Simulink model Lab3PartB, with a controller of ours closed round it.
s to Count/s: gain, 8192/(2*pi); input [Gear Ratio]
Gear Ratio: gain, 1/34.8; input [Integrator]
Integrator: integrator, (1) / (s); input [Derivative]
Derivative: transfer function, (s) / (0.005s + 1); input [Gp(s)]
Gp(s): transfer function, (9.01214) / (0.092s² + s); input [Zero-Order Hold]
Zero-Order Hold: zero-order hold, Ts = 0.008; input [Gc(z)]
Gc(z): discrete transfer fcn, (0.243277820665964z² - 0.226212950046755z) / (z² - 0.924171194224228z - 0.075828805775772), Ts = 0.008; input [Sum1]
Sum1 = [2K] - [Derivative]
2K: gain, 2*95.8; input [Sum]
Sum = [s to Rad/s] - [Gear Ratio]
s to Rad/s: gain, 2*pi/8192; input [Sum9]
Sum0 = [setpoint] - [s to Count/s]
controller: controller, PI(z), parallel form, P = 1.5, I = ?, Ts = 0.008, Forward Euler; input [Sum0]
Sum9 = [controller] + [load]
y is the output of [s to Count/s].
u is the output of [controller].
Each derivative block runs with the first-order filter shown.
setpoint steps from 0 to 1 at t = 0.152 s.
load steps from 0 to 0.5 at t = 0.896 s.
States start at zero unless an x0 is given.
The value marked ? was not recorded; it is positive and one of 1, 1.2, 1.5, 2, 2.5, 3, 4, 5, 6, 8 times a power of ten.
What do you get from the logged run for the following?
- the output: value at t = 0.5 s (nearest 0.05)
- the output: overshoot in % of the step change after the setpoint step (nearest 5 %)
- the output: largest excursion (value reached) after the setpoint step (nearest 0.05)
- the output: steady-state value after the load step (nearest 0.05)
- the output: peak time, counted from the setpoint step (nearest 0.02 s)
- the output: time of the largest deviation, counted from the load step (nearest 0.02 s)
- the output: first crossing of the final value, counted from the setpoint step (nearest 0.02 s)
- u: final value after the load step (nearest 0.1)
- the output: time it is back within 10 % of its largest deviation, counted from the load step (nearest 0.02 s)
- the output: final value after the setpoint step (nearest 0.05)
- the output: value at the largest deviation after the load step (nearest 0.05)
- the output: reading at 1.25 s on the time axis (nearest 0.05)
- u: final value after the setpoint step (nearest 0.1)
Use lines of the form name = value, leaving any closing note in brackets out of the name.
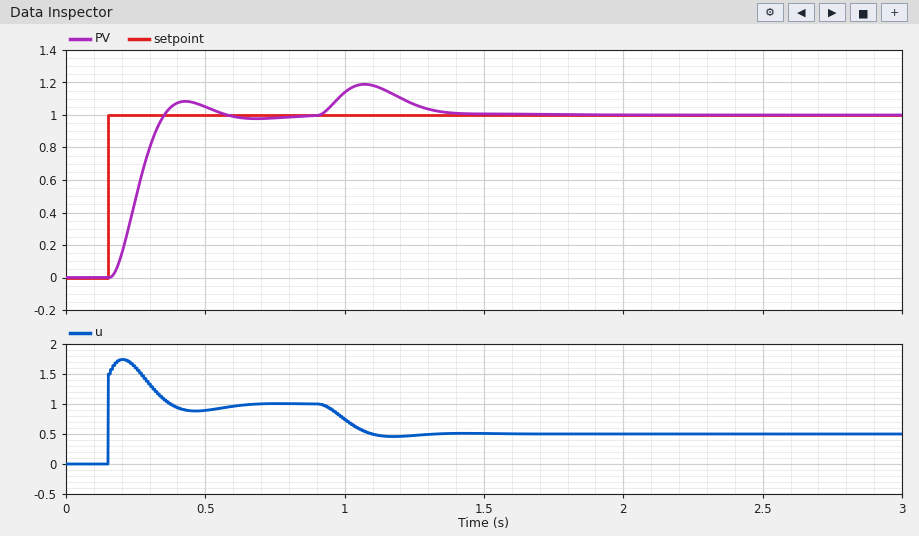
the output: value at t = 0.5 s = 1.05
the output: overshoot in % of the step change after the setpoint step = 10 %
the output: largest excursion (value reached) after the setpoint step = 1.10
the output: steady-state value after the load step = 1.00
the output: peak time, counted from the setpoint step = 0.28 s
the output: time of the largest deviation, counted from the load step = 0.18 s
the output: first crossing of the final value, counted from the setpoint step = 0.20 s
u: final value after the load step = 0.5
the output: time it is back within 10 % of its largest deviation, counted from the load step = 0.46 s
the output: final value after the setpoint step = 1.00
the output: value at the largest deviation after the load step = 1.20
the output: reading at 1.25 s on the time axis = 1.05
u: final value after the setpoint step = 1.0
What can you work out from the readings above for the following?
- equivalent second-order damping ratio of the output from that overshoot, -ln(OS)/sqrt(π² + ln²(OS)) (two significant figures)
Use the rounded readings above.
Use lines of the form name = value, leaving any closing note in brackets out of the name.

equivalent second-order damping ratio of the output from that overshoot, -ln(OS)/sqrt(π² + ln²(OS)) = 0.59
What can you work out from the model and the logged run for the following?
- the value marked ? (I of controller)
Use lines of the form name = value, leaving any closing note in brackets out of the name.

the value marked ? = 10
